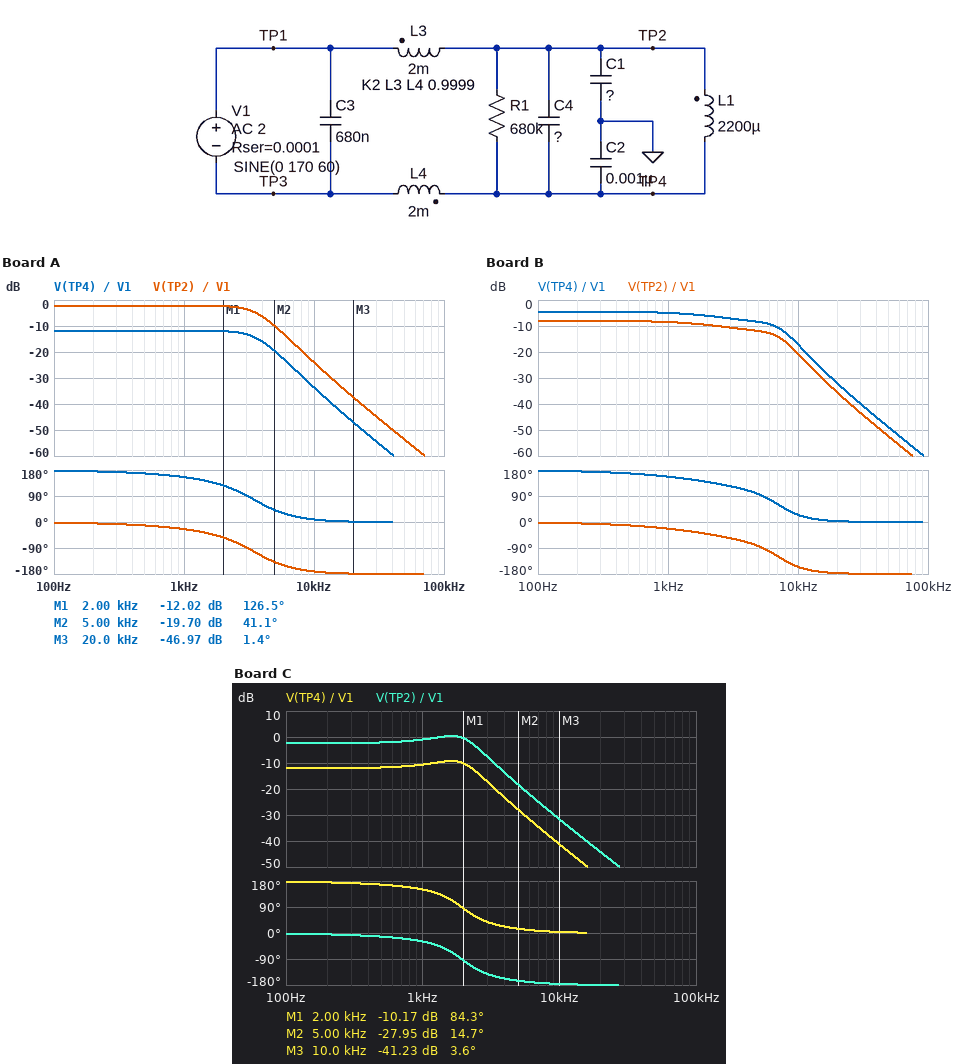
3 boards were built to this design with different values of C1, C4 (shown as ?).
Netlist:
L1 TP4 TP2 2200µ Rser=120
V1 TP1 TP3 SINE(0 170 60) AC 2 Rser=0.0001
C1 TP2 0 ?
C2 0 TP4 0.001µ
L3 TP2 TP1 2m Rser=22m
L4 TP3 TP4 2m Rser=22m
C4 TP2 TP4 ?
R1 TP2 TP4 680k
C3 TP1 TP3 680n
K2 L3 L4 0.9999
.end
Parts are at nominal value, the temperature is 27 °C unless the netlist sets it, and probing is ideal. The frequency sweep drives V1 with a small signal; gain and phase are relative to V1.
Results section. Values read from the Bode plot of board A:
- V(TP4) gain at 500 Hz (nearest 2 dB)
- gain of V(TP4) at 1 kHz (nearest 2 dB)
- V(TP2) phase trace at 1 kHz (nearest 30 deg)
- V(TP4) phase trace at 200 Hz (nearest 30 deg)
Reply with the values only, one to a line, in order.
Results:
-12 dB
-12 dB
-30 deg
180 deg
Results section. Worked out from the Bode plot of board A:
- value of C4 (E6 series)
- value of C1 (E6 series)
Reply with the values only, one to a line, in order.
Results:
470 nF
330 pF
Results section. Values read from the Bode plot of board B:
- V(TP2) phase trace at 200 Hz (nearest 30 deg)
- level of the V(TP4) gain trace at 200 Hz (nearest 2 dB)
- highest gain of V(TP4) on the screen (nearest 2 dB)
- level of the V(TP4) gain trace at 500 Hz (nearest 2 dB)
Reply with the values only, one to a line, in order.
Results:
0 deg
-4 dB
-4 dB
-4 dB
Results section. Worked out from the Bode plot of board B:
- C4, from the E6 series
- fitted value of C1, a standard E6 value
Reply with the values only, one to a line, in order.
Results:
220 nF
1.5 nF
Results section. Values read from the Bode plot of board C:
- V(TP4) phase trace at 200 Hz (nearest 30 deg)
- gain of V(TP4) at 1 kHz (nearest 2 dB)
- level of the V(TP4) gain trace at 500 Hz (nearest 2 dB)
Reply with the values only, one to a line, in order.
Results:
180 deg
-10 dB
-12 dB
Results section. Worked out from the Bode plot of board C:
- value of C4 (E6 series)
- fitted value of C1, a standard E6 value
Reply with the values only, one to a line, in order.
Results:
1 µF
330 pF
